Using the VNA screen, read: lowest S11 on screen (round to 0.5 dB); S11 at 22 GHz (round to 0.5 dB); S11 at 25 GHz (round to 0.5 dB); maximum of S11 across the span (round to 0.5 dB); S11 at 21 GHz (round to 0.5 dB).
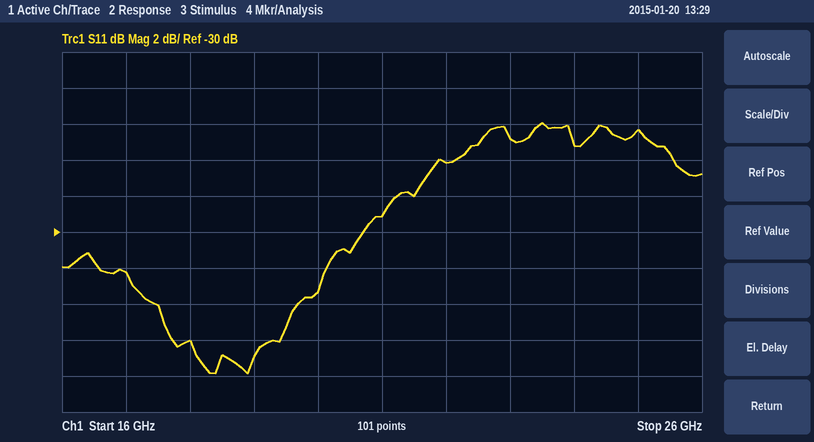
-38.0 dB
-26.0 dB
-24.5 dB
-24.0 dB
-29.0 dB
